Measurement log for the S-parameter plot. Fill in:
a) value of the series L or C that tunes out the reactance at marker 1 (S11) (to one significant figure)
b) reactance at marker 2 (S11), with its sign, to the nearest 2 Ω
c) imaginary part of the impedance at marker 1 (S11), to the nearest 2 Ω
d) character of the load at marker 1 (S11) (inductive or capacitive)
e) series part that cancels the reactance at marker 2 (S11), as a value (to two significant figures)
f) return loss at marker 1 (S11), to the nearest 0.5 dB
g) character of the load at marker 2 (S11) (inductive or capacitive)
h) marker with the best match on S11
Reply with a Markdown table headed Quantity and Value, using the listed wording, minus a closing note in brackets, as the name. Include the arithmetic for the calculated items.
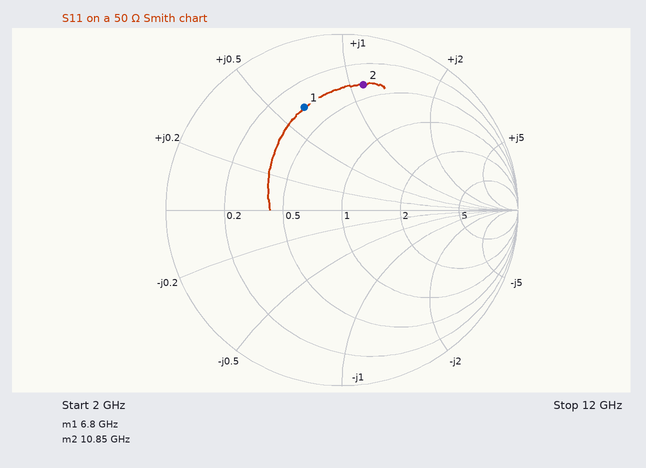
| Quantity | Value |
|---|---|
| value of the series L or C that tunes out the reactance at marker 1 (S11) | C = 1/(2π × 6.8 GHz × 32 Ω) ≈ 731 fF, so 700 fF to one significant figure |
| reactance at marker 2 (S11), with its sign, to the nearest 2 Ω | +56 Ω |
| imaginary part of the impedance at marker 1 (S11), to the nearest 2 Ω | +32 Ω |
| character of the load at marker 1 (S11) | inductive |
| series part that cancels the reactance at marker 2 (S11), as a value | C = 1/(2π × 10.85 GHz × 56 Ω) ≈ 262 fF, so 260 fF to two significant figures |
| return loss at marker 1 (S11), to the nearest 0.5 dB | 4.0 dB |
| character of the load at marker 2 (S11) | inductive |
| marker with the best match on S11 | marker 1 |
